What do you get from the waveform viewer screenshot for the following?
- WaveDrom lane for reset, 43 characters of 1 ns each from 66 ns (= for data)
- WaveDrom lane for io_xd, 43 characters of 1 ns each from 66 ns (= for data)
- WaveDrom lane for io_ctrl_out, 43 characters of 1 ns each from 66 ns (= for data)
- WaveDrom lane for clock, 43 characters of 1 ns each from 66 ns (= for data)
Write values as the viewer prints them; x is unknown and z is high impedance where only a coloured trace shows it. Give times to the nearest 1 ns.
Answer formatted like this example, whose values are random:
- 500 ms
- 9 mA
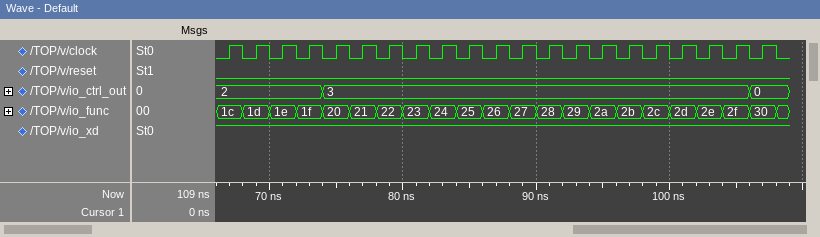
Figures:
- {name: 'reset', wave: '0..........................................'}
- {name: 'io_xd', wave: '1..........................................'}
- {name: 'io_ctrl_out', wave: '=.......=...............................=..', data: '2 3 0'}
- {name: 'clock', wave: '0101010101010101010101010101010101010101010'}
